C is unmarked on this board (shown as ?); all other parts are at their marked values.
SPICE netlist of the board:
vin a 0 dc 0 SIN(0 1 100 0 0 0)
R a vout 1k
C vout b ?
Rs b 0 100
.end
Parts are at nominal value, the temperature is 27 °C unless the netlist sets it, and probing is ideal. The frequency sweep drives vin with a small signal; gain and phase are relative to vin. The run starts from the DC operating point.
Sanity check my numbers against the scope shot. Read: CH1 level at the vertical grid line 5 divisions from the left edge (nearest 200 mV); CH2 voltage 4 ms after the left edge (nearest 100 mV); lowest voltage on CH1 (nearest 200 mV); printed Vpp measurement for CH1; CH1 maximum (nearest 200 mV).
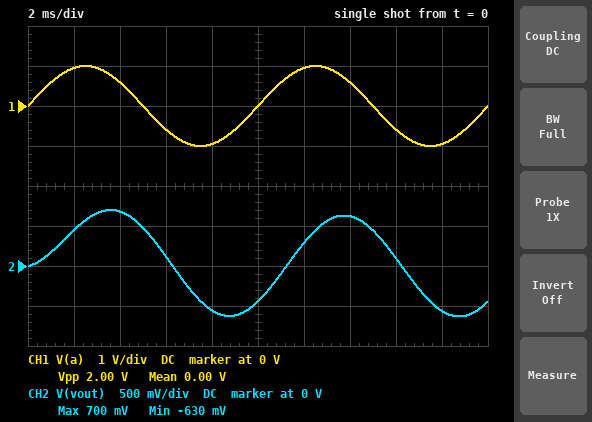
0 V
700 mV
-1.0 V
2.00 V
1.0 V
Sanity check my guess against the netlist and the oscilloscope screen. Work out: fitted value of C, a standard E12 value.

1.8 µF
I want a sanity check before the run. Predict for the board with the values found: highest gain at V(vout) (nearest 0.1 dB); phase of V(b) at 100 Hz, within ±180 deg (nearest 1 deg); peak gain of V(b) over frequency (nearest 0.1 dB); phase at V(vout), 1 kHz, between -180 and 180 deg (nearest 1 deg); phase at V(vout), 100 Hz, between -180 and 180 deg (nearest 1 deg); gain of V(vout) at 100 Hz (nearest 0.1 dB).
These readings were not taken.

0 dB
39 deg
-20.8 dB
-37 deg
-45 deg
-4.0 dB
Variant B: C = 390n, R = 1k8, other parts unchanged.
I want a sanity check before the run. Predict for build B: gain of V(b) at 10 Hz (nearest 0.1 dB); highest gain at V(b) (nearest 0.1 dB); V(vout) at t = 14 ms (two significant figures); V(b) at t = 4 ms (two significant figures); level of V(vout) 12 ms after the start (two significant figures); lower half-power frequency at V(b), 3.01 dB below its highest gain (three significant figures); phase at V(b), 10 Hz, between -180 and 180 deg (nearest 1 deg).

-52.2 dB
-25.6 dB
780 mV
-11 mV
680 mV
215 Hz
87 deg
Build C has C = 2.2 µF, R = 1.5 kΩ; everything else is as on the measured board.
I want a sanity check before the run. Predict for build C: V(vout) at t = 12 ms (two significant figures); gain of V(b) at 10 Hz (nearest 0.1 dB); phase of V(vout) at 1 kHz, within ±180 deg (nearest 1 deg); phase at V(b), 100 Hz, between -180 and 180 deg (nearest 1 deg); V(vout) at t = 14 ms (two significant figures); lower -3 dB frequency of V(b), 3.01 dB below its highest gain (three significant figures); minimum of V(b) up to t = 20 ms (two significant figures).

110 mV
-37.4 dB
-33 deg
24 deg
420 mV
45.2 Hz
-60 mV
